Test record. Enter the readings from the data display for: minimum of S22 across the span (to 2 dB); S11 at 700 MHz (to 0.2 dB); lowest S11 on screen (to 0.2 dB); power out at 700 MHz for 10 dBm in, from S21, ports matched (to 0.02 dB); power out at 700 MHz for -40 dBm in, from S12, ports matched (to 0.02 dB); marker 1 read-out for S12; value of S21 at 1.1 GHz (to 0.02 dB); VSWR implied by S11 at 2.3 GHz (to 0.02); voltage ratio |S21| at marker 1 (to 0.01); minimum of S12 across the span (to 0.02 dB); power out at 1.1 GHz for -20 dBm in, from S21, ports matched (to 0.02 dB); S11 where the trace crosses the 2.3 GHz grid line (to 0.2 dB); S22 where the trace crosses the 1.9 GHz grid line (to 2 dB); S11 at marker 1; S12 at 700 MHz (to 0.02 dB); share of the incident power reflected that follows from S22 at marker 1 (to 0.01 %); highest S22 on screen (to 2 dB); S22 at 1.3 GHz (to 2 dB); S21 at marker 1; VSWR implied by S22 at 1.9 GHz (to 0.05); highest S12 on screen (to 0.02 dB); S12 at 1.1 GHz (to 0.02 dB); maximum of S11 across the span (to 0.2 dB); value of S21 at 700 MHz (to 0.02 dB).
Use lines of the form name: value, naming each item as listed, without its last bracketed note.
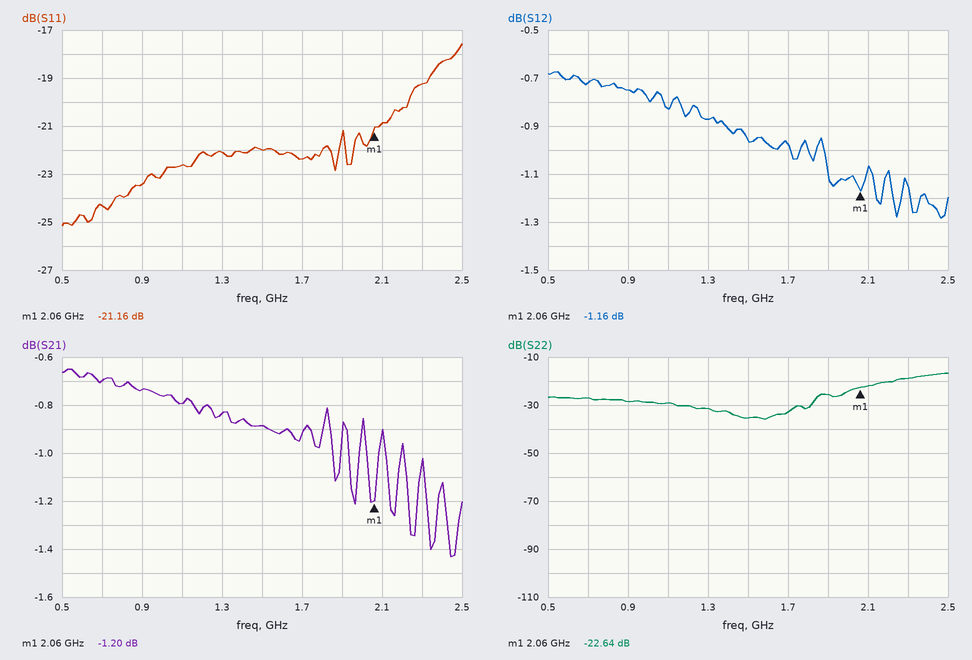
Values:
minimum of S22 across the span: -36 dB
S11 at 700 MHz: -24.4 dB
lowest S11 on screen: -25.2 dB
power out at 700 MHz for 10 dBm in, from S21, ports matched: 9.30 dBm
power out at 700 MHz for -40 dBm in, from S12, ports matched: -40.72 dBm
marker 1 read-out for S12: -1.16 dB
value of S21 at 1.1 GHz: -0.80 dB
VSWR implied by S11 at 2.3 GHz: 1.24
voltage ratio |S21| at marker 1: 0.87
minimum of S12 across the span: -1.28 dB
power out at 1.1 GHz for -20 dBm in, from S21, ports matched: -20.80 dBm
S11 where the trace crosses the 2.3 GHz grid line: -19.2 dB
S22 where the trace crosses the 1.9 GHz grid line: -26 dB
S11 at marker 1: -21.16 dB
S12 at 700 MHz: -0.72 dB
share of the incident power reflected that follows from S22 at marker 1: 0.54 %
highest S22 on screen: -16 dB
S22 at 1.3 GHz: -32 dB
S21 at marker 1: -1.20 dB
VSWR implied by S22 at 1.9 GHz: 1.10
highest S12 on screen: -0.68 dB
S12 at 1.1 GHz: -0.82 dB
maximum of S11 across the span: -17.6 dB
value of S21 at 700 MHz: -0.70 dB
